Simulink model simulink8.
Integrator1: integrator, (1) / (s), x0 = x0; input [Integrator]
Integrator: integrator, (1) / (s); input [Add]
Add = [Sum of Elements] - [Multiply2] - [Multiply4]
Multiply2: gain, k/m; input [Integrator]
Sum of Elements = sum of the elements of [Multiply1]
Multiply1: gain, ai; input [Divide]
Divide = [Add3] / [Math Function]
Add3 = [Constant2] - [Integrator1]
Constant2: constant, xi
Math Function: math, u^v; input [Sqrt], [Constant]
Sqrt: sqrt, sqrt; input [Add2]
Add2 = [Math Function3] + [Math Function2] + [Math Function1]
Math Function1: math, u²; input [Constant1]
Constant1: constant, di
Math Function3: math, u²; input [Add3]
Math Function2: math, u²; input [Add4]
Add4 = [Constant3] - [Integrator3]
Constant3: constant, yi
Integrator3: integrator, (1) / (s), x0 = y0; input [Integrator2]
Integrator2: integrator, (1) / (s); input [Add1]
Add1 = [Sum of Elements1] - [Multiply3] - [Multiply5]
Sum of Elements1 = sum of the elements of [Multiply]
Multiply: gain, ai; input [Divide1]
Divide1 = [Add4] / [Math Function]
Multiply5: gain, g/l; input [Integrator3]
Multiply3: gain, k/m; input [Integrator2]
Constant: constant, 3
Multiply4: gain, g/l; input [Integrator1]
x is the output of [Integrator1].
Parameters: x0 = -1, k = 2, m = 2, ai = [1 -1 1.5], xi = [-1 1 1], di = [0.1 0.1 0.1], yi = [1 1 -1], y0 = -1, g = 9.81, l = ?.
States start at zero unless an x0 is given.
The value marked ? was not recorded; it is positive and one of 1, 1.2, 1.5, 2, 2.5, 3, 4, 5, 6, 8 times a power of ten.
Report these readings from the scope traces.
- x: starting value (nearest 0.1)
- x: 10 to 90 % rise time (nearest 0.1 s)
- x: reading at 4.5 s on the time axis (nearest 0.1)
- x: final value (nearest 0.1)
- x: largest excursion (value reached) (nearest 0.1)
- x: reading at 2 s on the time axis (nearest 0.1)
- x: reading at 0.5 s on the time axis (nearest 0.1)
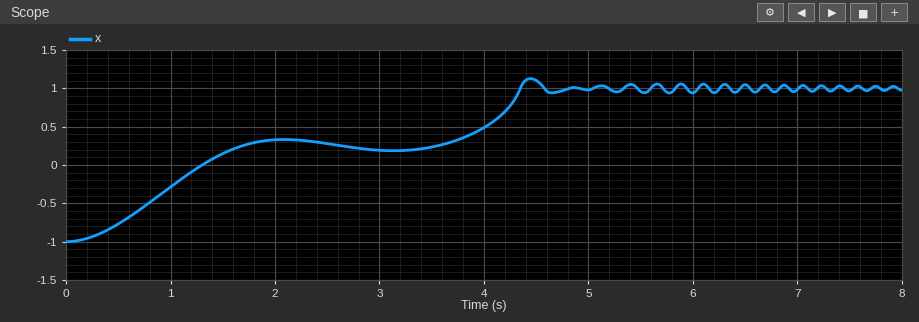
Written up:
-1.0
3.8 s
1.1
1.0
1.1
0.3
-0.8
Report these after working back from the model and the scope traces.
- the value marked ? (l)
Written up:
5
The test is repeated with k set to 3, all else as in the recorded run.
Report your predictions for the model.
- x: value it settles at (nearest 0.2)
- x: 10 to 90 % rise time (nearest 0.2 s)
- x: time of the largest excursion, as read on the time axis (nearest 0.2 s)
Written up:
1.0
4.4 s
5.2 s
